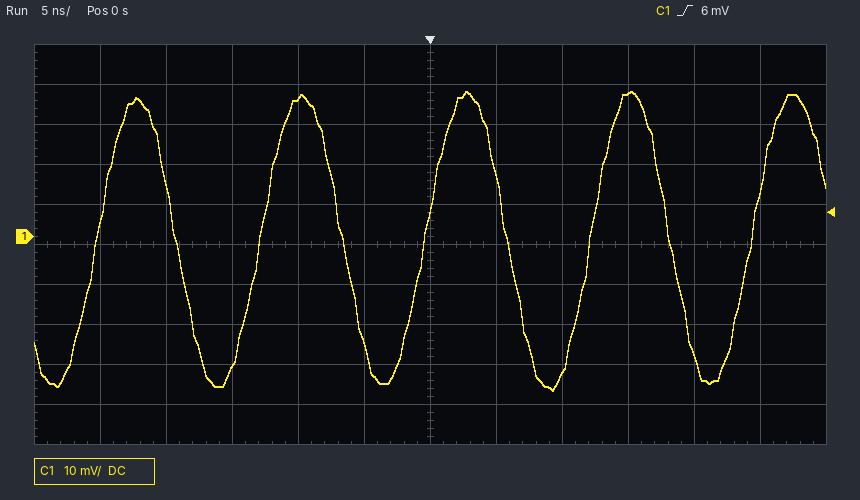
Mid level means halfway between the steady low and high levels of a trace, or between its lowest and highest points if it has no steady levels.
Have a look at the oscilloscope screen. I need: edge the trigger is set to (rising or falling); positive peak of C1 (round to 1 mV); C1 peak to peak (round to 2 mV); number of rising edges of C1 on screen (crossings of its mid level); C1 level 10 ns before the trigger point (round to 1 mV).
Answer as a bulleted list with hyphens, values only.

- rising
- 36 mV
- 74 mV
- 5
- 35 mV
